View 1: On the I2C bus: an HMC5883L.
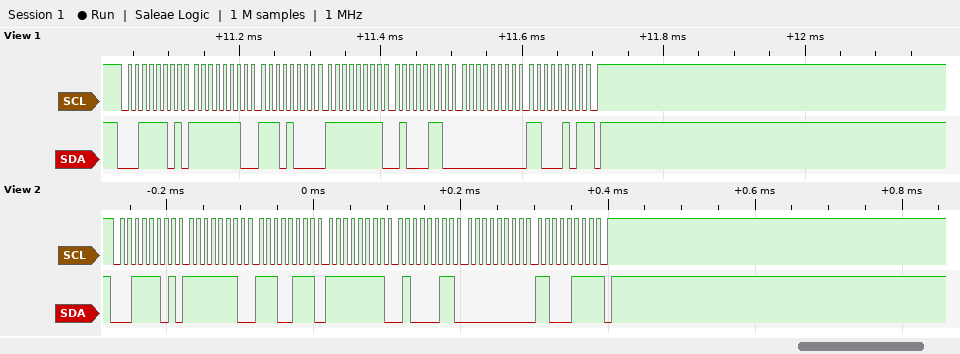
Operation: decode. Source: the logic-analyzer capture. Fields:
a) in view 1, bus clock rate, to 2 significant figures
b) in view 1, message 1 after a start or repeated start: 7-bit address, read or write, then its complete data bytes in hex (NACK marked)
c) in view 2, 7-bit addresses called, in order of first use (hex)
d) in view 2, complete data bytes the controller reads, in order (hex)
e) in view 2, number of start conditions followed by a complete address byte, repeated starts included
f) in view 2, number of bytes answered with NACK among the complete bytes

100 kHz
0x1E read: FE E8 FF 46 00 C5 NACK
0x1E
FE E7 FF 43 00 C7
1
1
